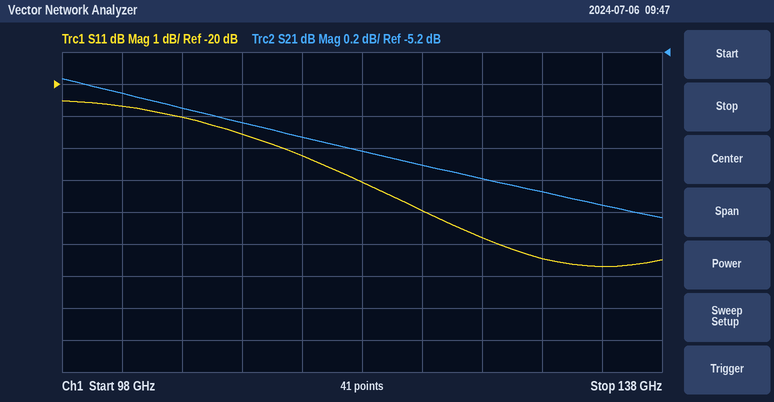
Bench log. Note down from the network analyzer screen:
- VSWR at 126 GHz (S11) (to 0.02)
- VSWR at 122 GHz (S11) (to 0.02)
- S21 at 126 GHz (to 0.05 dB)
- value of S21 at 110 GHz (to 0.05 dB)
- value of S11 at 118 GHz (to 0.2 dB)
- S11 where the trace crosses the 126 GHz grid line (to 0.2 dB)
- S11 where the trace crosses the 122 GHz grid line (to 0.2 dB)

1.12
1.14
-6.00 dB
-5.65 dB
-23.0 dB
-24.8 dB
-24.0 dB
